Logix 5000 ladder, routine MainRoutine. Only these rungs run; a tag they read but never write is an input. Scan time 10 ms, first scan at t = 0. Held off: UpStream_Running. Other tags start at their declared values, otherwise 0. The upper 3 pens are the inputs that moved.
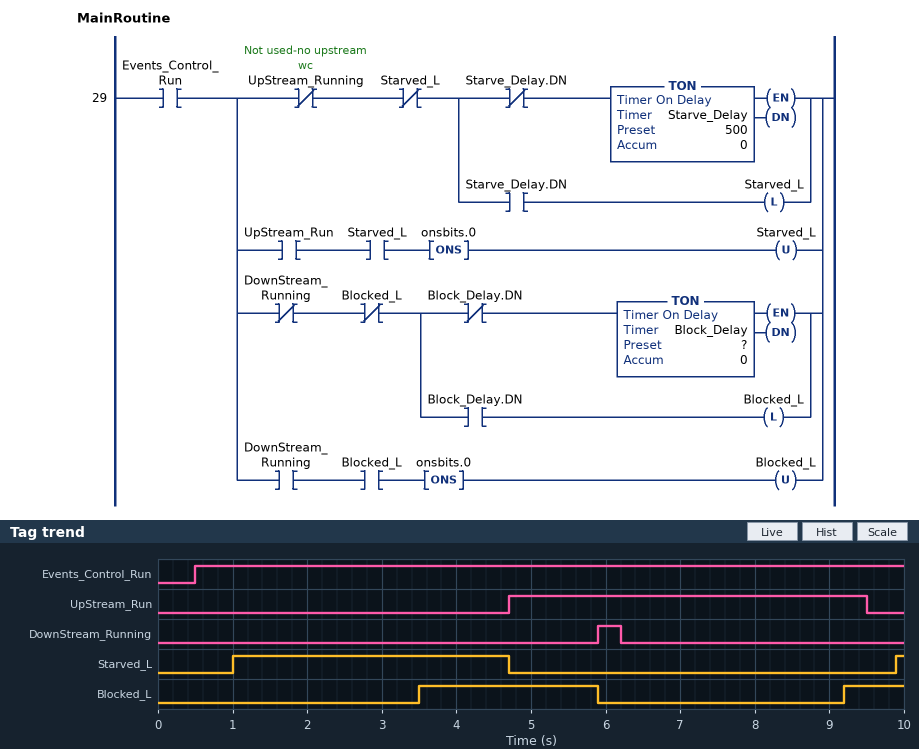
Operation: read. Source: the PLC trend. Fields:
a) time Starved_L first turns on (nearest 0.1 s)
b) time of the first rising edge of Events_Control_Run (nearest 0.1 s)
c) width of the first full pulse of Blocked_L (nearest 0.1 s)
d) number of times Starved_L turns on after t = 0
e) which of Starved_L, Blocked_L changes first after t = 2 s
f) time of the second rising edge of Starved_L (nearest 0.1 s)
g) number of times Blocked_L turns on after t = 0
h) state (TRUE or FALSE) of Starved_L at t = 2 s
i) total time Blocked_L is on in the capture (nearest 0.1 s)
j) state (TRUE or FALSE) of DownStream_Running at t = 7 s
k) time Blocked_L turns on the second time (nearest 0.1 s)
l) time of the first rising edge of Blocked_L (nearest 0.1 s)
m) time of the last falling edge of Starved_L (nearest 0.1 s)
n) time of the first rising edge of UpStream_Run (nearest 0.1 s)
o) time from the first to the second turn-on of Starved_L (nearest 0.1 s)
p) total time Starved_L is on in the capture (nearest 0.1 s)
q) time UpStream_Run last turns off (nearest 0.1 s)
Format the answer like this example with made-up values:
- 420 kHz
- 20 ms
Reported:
- 1.0 s
- 0.5 s
- 2.4 s
- 2
- Blocked_L
- 9.9 s
- 2
- TRUE
- 3.2 s
- FALSE
- 9.2 s
- 3.5 s
- 4.7 s
- 4.7 s
- 8.9 s
- 3.8 s
- 9.5 s
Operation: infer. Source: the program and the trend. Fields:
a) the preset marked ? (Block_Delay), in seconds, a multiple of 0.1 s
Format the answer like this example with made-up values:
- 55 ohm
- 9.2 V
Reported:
- 3.0 s
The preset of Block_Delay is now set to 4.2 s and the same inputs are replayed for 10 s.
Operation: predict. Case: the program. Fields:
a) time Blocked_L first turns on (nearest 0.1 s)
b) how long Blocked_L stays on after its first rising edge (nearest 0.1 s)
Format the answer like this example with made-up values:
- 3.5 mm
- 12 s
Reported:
- 4.7 s
- 1.2 s
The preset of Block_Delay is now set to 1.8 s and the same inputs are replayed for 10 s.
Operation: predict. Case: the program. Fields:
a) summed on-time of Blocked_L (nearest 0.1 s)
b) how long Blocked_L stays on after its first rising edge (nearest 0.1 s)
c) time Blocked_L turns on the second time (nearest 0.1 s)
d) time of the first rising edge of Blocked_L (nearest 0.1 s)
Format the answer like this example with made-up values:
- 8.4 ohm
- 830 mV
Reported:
- 5.6 s
- 3.6 s
- 8.0 s
- 2.3 s
